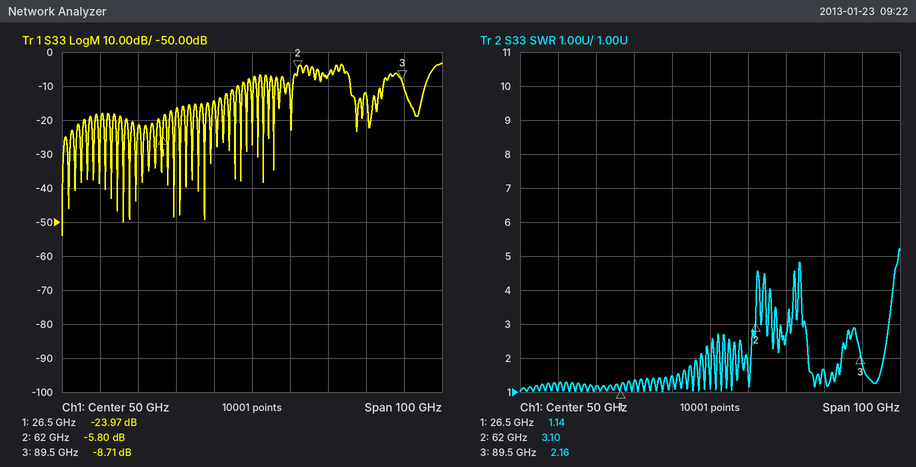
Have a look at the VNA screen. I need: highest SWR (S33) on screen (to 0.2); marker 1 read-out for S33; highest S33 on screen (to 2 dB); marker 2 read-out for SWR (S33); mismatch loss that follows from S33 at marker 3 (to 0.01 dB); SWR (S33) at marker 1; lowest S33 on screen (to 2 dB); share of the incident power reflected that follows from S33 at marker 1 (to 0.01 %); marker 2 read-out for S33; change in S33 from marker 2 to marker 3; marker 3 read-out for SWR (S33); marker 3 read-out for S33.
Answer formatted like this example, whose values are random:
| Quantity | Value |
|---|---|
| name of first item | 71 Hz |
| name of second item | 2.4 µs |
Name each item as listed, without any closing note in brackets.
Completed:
| Quantity | Value |
|---|---|
| highest SWR (S33) on screen | 5.2 |
| marker 1 read-out for S33 | -23.97 dB |
| highest S33 on screen | -4 dB |
| marker 2 read-out for SWR | 3.10 |
| mismatch loss that follows from S33 at marker 3 | 0.63 dB |
| SWR (S33) at marker 1 | 1.14 |
| lowest S33 on screen | -54 dB |
| share of the incident power reflected that follows from S33 at marker 1 | 0.40 % |
| marker 2 read-out for S33 | -5.80 dB |
| change in S33 from marker 2 to marker 3 | -2.91 dB |
| marker 3 read-out for SWR | 2.16 |
| marker 3 read-out for S33 | -8.71 dB |
